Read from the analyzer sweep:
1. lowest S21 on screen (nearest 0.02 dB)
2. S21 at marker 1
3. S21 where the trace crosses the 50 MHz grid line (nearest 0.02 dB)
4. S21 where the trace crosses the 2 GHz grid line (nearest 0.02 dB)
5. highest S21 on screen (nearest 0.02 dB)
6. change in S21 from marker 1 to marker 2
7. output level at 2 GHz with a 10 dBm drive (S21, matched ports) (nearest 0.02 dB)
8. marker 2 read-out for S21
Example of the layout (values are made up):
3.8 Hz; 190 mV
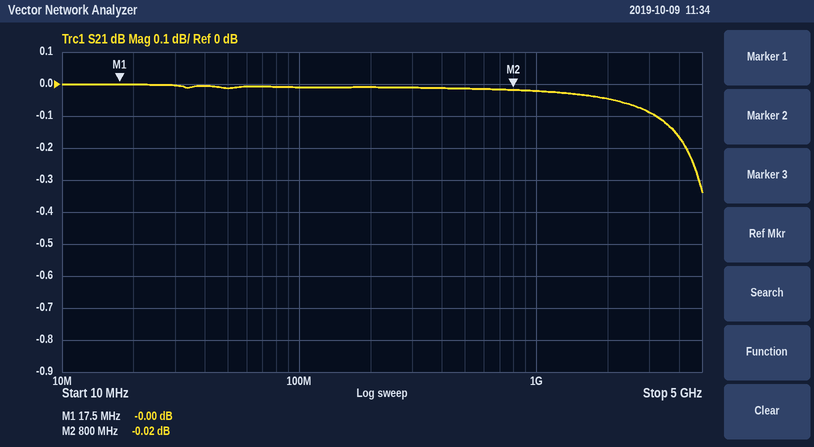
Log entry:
-0.34 dB; -0.00 dB; -0.02 dB; -0.04 dB; 0.00 dB; -0.02 dB; 9.96 dBm; -0.02 dB
